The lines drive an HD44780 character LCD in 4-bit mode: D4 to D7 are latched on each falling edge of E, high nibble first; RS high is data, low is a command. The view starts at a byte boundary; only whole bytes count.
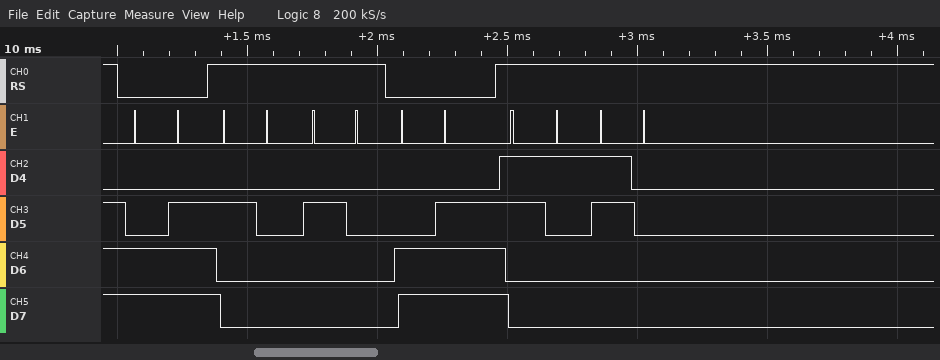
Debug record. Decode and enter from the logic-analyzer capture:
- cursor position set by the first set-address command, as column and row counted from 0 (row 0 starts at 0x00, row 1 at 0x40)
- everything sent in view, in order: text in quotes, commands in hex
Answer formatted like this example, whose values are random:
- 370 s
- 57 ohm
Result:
- column 14, row 1
- 0xCE "  " 0xCE "10"
